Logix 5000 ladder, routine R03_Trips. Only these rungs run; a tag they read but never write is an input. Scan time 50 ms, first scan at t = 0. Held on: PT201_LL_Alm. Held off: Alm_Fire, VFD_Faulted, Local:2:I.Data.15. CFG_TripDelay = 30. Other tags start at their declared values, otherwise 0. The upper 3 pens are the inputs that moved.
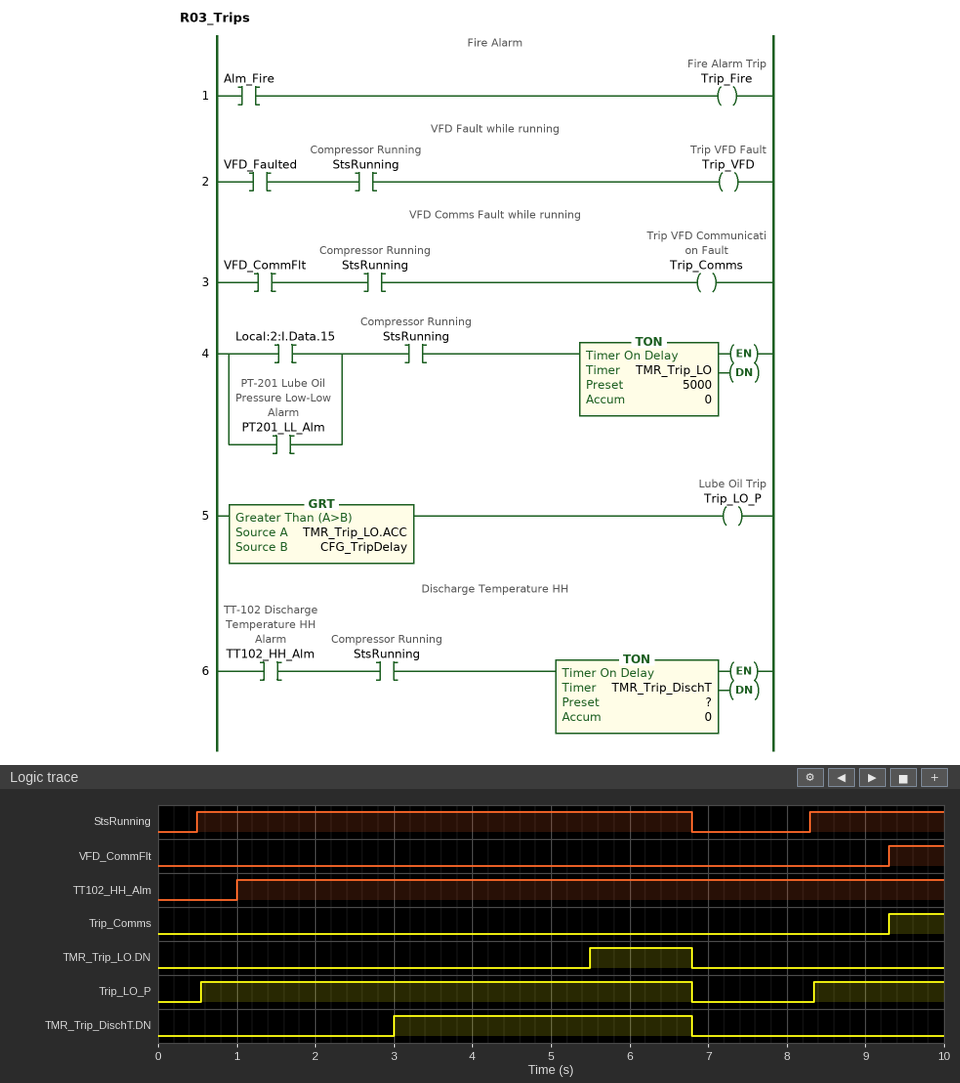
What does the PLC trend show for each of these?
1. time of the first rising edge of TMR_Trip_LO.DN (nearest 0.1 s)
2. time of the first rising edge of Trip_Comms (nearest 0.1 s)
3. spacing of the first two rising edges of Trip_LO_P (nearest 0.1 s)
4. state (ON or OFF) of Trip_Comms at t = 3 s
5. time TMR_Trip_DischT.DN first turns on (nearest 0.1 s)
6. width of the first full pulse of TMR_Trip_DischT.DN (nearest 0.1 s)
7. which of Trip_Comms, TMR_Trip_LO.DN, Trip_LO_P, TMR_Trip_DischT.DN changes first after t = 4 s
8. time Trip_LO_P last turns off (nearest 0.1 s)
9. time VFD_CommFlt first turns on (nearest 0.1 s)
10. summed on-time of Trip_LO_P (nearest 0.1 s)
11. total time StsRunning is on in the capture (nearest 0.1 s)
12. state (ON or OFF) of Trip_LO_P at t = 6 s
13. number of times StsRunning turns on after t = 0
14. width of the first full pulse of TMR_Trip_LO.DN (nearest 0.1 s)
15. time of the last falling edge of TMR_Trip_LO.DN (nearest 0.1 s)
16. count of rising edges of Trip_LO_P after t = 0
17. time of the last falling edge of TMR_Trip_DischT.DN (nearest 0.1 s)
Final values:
5.5 s
9.3 s
7.8 s
OFF
3.0 s
3.8 s
TMR_Trip_LO.DN
6.8 s
9.3 s
7.9 s
8.0 s
ON
2
1.3 s
6.8 s
2
6.8 s
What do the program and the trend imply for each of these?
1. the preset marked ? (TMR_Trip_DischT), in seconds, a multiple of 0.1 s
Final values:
2.0 s
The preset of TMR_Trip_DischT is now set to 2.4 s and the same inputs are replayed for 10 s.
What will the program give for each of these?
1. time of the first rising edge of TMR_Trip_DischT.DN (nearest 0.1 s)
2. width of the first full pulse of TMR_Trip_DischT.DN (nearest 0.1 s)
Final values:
3.4 s
3.4 s
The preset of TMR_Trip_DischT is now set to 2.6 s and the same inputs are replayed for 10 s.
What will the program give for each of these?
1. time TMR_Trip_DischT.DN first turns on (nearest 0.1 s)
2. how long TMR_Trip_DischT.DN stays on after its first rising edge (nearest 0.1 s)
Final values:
3.6 s
3.2 s
